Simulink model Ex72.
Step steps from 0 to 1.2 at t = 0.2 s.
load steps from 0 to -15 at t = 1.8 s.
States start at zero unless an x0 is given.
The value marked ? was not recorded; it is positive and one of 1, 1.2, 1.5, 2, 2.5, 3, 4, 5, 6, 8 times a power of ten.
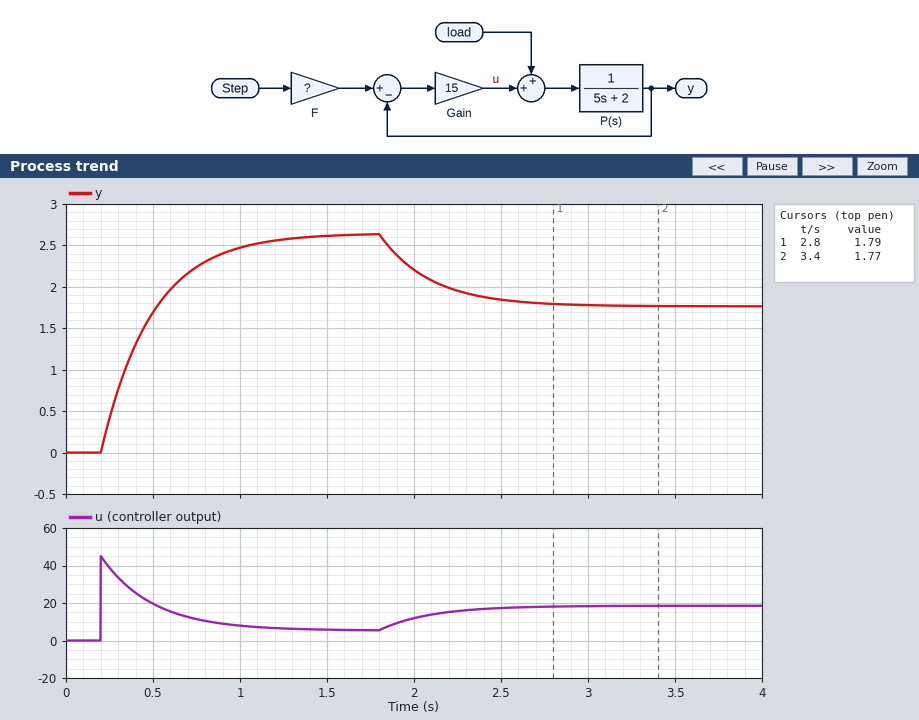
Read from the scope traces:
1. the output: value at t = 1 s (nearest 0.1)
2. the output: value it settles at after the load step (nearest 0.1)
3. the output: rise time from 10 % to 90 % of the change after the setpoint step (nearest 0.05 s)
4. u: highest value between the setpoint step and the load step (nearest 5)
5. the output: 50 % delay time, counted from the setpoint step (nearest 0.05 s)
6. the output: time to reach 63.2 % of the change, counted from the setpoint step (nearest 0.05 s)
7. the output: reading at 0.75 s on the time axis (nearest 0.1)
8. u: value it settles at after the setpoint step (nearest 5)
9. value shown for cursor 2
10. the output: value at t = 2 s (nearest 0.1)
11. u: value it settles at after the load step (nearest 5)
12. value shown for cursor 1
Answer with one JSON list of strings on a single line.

["2.5", "1.8", "0.65 s", "45", "0.20 s", "0.30 s", "2.2", "5", "1.77", "2.2", "20", "1.79"]
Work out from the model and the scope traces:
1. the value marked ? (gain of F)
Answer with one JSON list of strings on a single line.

["2.5"]
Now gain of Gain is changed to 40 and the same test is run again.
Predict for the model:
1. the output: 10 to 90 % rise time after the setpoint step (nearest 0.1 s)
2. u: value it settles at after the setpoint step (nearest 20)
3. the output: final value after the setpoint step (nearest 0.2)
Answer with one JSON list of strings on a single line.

["0.3 s", "0", "2.8"]
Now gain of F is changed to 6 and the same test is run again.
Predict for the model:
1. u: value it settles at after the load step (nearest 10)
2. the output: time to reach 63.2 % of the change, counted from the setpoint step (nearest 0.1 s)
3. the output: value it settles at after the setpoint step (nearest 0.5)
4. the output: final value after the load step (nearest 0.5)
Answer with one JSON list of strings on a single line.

["30", "0.3 s", "6.5", "5.5"]
